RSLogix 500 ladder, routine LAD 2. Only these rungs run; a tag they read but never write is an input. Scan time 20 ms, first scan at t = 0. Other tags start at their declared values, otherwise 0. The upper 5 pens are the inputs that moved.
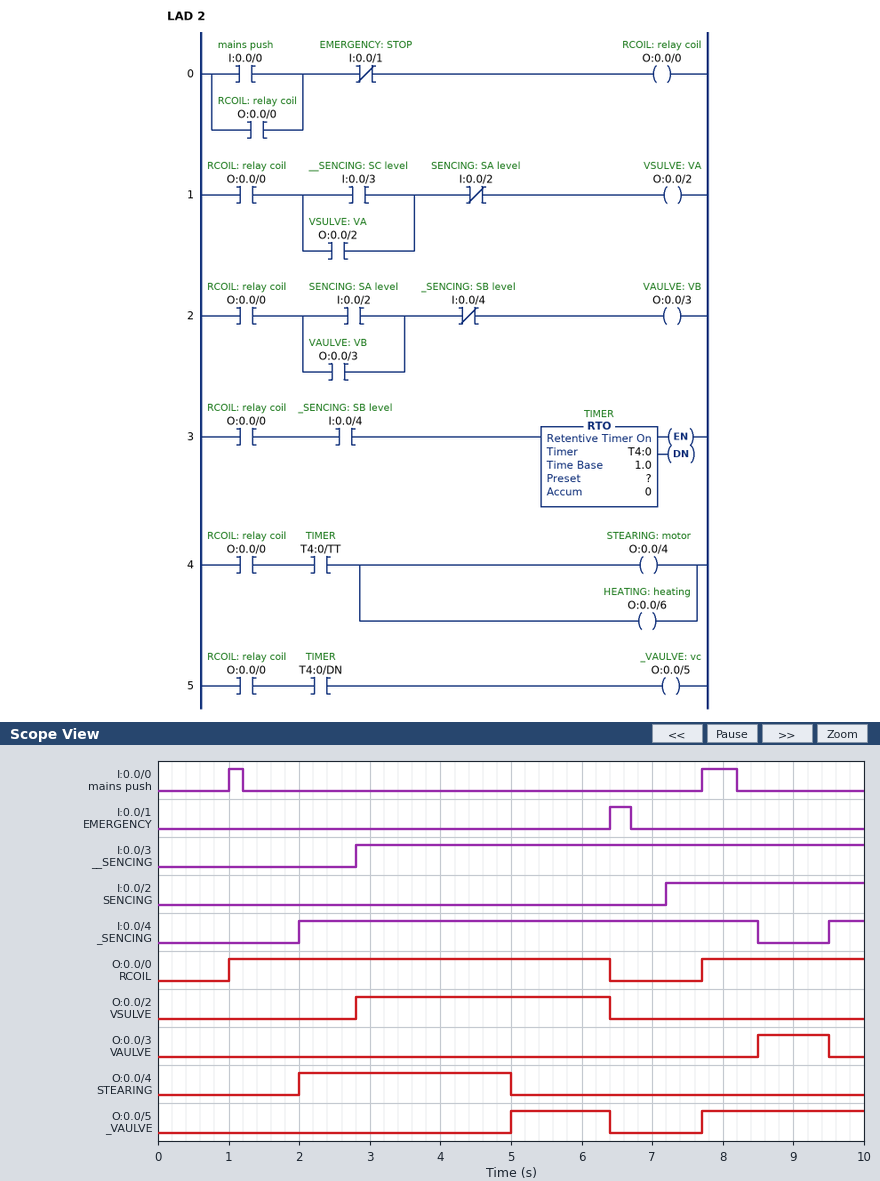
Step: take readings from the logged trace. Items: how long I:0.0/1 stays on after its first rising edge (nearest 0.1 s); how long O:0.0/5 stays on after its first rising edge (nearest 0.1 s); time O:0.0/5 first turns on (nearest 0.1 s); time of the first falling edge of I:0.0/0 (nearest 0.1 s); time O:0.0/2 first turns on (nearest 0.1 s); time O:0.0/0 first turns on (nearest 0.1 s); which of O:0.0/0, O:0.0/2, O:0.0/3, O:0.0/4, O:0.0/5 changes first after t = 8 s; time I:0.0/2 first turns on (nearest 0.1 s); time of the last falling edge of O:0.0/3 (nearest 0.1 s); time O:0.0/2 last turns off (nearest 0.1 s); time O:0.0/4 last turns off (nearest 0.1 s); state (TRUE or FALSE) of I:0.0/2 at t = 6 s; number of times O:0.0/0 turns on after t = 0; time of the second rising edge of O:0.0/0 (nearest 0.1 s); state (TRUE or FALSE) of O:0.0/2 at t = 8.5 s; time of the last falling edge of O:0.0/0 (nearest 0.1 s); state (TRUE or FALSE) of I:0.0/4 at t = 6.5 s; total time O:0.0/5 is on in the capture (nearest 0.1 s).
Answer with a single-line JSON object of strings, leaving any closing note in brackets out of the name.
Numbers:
{"how long I:0.0/1 stays on after its first rising edge": "0.3 s", "how long O:0.0/5 stays on after its first rising edge": "1.4 s", "time O:0.0/5 first turns on": "5.0 s", "time of the first falling edge of I:0.0/0": "1.2 s", "time O:0.0/2 first turns on": "2.8 s", "time O:0.0/0 first turns on": "1.0 s", "which of O:0.0/0, O:0.0/2, O:0.0/3, O:0.0/4, O:0.0/5 changes first after t = 8 s": "O:0.0/3", "time I:0.0/2 first turns on": "7.2 s", "time of the last falling edge of O:0.0/3": "9.5 s", "time O:0.0/2 last turns off": "6.4 s", "time O:0.0/4 last turns off": "5.0 s", "state (TRUE or FALSE) of I:0.0/2 at t = 6 s": "FALSE", "number of times O:0.0/0 turns on after t = 0": "2", "time of the second rising edge of O:0.0/0": "7.7 s", "state (TRUE or FALSE) of O:0.0/2 at t = 8.5 s": "FALSE", "time of the last falling edge of O:0.0/0": "6.4 s", "state (TRUE or FALSE) of I:0.0/4 at t = 6.5 s": "TRUE", "total time O:0.0/5 is on in the capture": "3.7 s"}
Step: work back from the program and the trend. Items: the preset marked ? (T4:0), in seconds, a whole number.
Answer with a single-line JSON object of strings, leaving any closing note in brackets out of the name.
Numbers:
{"the preset marked ? (T4:0), in seconds, a whole number": "3 s"}
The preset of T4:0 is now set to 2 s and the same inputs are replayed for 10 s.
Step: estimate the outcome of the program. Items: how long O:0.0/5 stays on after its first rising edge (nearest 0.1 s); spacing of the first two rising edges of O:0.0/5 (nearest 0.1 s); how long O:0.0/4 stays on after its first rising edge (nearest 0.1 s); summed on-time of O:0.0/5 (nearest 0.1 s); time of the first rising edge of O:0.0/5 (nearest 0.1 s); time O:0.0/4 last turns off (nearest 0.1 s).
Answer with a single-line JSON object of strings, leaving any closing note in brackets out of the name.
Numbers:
{"how long O:0.0/5 stays on after its first rising edge": "2.4 s", "spacing of the first two rising edges of O:0.0/5": "3.7 s", "how long O:0.0/4 stays on after its first rising edge": "2.0 s", "summed on-time of O:0.0/5": "4.7 s", "time of the first rising edge of O:0.0/5": "4.0 s", "time O:0.0/4 last turns off": "4.0 s"}
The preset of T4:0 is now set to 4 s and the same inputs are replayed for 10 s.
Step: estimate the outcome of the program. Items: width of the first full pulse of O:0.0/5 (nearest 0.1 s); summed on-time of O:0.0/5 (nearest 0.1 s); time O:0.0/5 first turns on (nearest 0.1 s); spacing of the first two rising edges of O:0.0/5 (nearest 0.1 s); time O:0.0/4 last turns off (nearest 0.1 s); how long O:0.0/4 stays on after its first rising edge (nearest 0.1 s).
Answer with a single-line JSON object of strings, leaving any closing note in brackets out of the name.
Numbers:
{"width of the first full pulse of O:0.0/5": "0.4 s", "summed on-time of O:0.0/5": "2.7 s", "time O:0.0/5 first turns on": "6.0 s", "spacing of the first two rising edges of O:0.0/5": "1.7 s", "time O:0.0/4 last turns off": "6.0 s", "how long O:0.0/4 stays on after its first rising edge": "4.0 s"}
